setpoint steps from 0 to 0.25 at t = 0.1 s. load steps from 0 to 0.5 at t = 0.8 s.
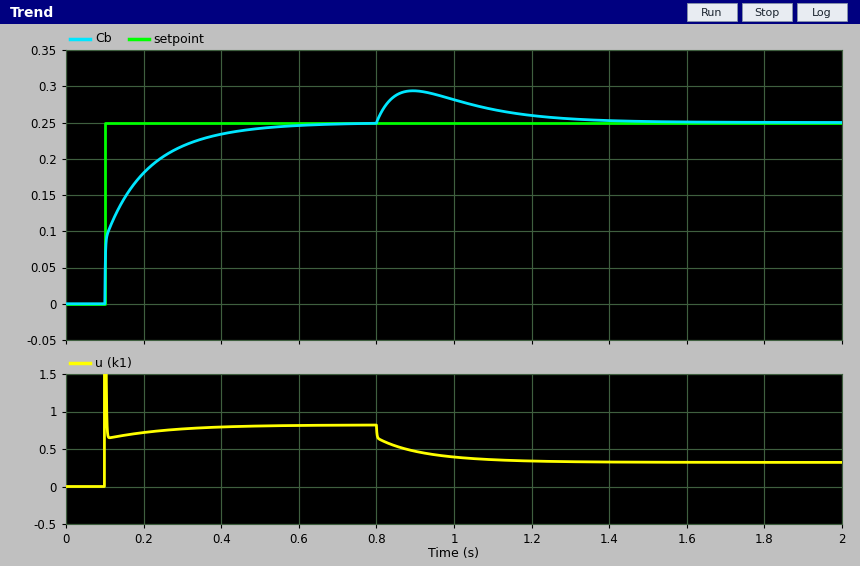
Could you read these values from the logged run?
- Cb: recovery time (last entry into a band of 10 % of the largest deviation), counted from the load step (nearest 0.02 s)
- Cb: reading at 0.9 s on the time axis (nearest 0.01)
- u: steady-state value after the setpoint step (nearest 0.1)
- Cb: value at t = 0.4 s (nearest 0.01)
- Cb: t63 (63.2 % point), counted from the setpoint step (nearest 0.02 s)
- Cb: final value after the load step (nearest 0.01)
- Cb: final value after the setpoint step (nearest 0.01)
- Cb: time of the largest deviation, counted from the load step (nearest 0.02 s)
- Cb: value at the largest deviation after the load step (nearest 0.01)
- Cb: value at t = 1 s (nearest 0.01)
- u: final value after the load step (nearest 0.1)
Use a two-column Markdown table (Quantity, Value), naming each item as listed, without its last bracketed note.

| Quantity | Value |
|---|---|
| Cb: recovery time (last entry into a band of 10 % of the largest deviation), counted from the load step | 0.52 s |
| Cb: reading at 0.9 s on the time axis | 0.29 |
| u: steady-state value after the setpoint step | 0.8 |
| Cb: value at t = 0.4 s | 0.23 |
| Cb: t63 (63.2 % point), counted from the setpoint step | 0.06 s |
| Cb: final value after the load step | 0.25 |
| Cb: final value after the setpoint step | 0.25 |
| Cb: time of the largest deviation, counted from the load step | 0.10 s |
| Cb: value at the largest deviation after the load step | 0.29 |
| Cb: value at t = 1 s | 0.28 |
| u: final value after the load step | 0.3 |
